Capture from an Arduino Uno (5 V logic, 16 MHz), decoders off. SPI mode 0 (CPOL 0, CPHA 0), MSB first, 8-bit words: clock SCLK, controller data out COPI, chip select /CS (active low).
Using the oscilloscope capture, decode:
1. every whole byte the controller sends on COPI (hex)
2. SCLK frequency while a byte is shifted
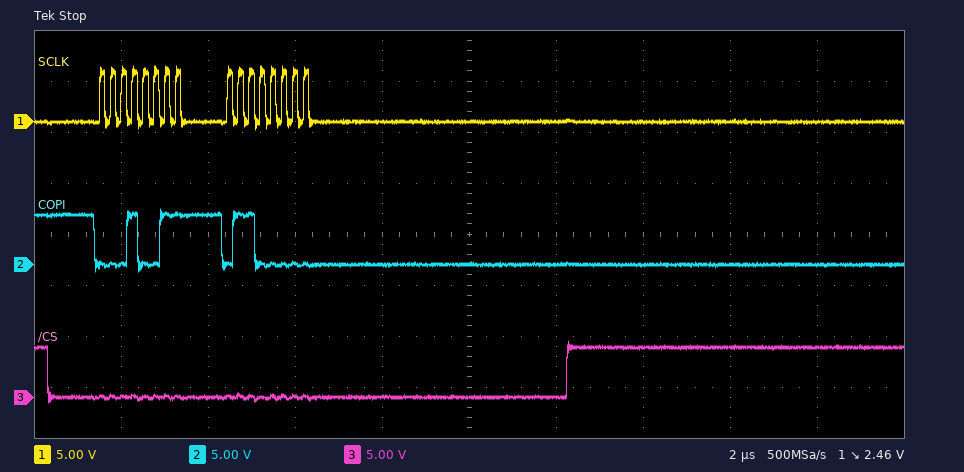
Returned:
0x13 0x60
4 MHz
